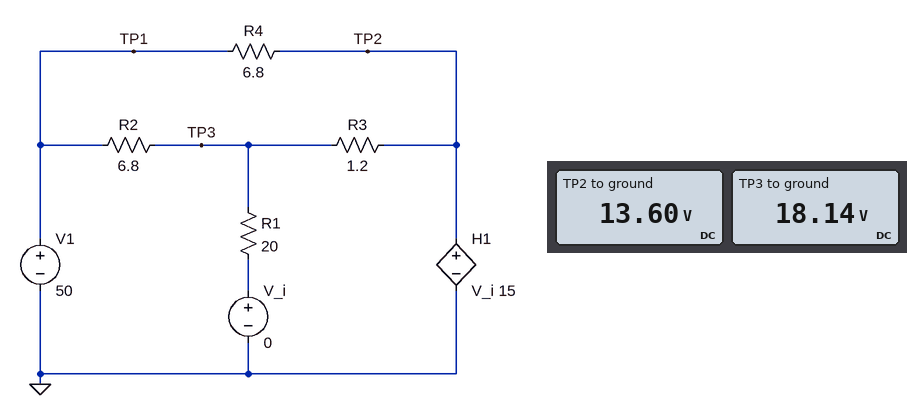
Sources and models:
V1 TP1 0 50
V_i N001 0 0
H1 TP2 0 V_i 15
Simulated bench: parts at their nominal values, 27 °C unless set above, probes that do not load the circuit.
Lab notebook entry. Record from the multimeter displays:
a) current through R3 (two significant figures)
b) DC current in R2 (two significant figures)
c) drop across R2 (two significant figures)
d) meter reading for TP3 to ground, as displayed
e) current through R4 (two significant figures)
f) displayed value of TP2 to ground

3.8 A
4.7 A
32 V
18.14 V
5.4 A
13.60 V
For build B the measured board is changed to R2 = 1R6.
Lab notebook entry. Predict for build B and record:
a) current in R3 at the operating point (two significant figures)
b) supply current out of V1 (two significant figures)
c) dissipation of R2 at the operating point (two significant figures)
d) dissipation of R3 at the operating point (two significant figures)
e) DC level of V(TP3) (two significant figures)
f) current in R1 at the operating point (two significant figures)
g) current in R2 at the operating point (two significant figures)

7.4 A
13 A
130 W
65 W
35 V
1.8 A
9.1 A
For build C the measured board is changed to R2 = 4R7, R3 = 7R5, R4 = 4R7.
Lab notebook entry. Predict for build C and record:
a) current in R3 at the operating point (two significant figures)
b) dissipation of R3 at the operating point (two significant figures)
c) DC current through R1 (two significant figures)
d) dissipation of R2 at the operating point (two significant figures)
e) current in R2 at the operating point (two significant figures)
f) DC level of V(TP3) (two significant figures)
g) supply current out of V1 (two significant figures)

1.2 A
11 W
1.8 A
42 W
3.0 A
36 V
7.9 A
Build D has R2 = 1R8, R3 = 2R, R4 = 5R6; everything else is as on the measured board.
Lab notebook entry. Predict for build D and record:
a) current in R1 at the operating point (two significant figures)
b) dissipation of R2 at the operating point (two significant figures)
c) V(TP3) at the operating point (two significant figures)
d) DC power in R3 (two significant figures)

1.9 A
80 W
38 V
45 W
